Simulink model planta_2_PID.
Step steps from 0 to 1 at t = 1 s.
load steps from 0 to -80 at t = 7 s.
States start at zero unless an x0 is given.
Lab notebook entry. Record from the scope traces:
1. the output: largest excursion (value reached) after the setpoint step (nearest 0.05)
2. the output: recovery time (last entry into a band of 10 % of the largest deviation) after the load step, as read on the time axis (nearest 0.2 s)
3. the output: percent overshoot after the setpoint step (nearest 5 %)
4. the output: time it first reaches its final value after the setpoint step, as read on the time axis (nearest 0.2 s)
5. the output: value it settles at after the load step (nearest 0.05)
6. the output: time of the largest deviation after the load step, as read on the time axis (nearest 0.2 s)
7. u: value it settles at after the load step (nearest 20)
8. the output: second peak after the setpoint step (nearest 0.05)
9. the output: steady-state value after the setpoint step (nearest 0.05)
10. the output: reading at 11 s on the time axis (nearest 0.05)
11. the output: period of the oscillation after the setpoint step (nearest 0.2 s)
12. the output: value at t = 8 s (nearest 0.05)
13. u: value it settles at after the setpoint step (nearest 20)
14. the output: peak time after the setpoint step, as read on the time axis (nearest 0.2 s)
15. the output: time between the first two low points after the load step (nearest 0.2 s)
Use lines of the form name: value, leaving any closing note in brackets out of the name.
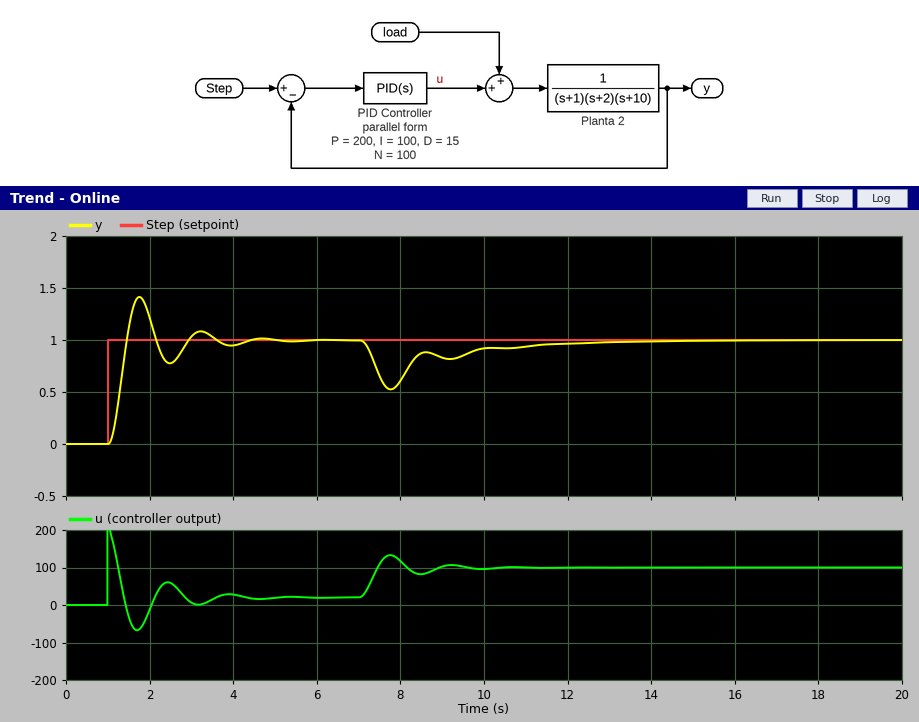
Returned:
the output: largest excursion (value reached) after the setpoint step: 1.40
the output: recovery time (last entry into a band of 10 % of the largest deviation) after the load step, as read on the time axis: 11.4 s
the output: percent overshoot after the setpoint step: 40 %
the output: time it first reaches its final value after the setpoint step, as read on the time axis: 1.4 s
the output: value it settles at after the load step: 1.00
the output: time of the largest deviation after the load step, as read on the time axis: 7.8 s
u: value it settles at after the load step: 100
the output: second peak after the setpoint step: 1.10
the output: steady-state value after the setpoint step: 1.00
the output: reading at 11 s on the time axis: 0.95
the output: period of the oscillation after the setpoint step: 1.4 s
the output: value at t = 8 s: 0.60
u: value it settles at after the setpoint step: 20
the output: peak time after the setpoint step, as read on the time axis: 1.8 s
the output: time between the first two low points after the load step: 1.4 s
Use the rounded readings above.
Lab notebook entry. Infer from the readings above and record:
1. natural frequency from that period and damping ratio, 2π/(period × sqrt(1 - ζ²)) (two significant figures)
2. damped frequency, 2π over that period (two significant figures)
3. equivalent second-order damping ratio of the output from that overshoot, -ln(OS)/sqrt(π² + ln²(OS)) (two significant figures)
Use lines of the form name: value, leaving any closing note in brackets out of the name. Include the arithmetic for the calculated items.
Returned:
natural frequency from that period and damping ratio, 2π/(period × sqrt(1 - ζ²)): 2π / (1.4 × sqrt(1 - 0.28²)) = 4.7 rad/s
damped frequency, 2π over that period: 2π / 1.4 = 4.5 rad/s
equivalent second-order damping ratio of the output from that overshoot, -ln(OS)/sqrt(π² + ln²(OS)): ln(0.4) = -0.916; 0.916 / sqrt(9.870 + 0.840) = 0.28
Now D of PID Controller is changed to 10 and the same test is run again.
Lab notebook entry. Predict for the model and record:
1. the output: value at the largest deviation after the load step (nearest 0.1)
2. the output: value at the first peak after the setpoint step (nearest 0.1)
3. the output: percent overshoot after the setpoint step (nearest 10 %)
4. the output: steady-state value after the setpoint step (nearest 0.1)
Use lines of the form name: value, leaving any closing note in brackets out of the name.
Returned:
the output: value at the largest deviation after the load step: 0.5
the output: value at the first peak after the setpoint step: 1.5
the output: percent overshoot after the setpoint step: 50 %
the output: steady-state value after the setpoint step: 1.0
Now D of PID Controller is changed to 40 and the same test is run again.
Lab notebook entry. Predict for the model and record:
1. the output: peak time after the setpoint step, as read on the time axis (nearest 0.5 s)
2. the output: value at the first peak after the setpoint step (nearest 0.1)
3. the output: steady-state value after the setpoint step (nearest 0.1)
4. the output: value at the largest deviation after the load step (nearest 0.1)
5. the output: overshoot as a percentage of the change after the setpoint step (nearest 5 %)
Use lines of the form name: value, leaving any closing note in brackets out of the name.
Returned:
the output: peak time after the setpoint step, as read on the time axis: 1.5 s
the output: value at the first peak after the setpoint step: 1.2
the output: steady-state value after the setpoint step: 1.0
the output: value at the largest deviation after the load step: 0.6
the output: overshoot as a percentage of the change after the setpoint step: 20 %
